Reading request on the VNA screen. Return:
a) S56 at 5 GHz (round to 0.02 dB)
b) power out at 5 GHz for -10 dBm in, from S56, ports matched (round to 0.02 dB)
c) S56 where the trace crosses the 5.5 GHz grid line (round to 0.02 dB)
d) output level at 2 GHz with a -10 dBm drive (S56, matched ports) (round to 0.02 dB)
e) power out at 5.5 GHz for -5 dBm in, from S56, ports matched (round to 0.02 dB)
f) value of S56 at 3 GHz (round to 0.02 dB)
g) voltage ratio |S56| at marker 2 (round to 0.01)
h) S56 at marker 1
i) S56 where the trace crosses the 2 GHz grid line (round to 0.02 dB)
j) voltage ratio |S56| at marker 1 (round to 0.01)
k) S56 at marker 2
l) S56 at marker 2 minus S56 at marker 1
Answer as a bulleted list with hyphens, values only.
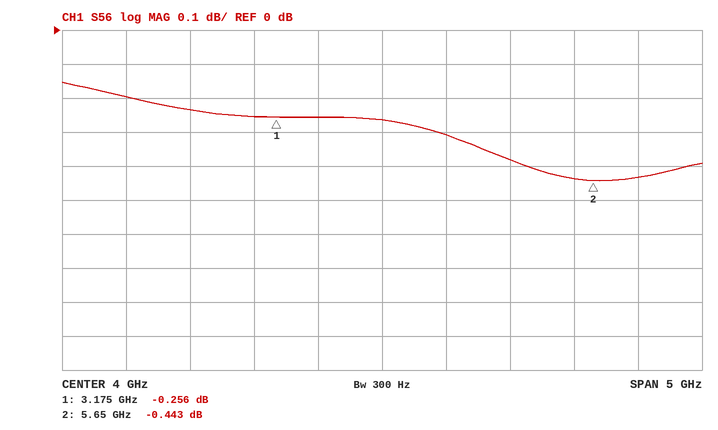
- -0.38 dB
- -10.38 dBm
- -0.44 dB
- -10.20 dBm
- -5.44 dBm
- -0.26 dB
- 0.95
- -0.256 dB
- -0.20 dB
- 0.97
- -0.443 dB
- -0.187 dB
